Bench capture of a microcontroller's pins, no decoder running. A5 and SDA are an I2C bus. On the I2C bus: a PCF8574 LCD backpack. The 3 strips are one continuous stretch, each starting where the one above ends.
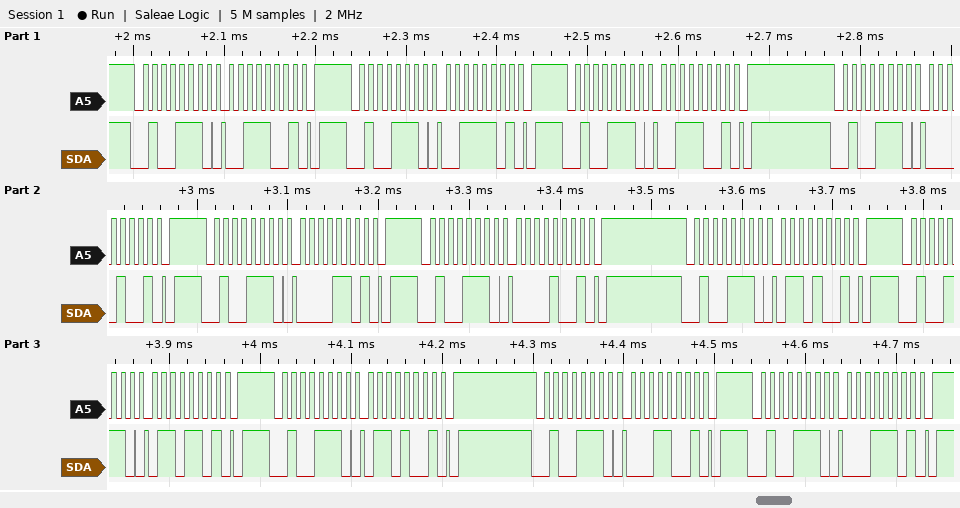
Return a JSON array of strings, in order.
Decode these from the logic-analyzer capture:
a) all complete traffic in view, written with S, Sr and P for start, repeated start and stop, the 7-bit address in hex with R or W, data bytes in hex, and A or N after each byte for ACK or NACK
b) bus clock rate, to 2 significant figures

["S 27W A 39 A P S 27W A 3D A P S 27W A 39 A P S 27W A 09 A P S 27W A 0D A P S 27W A 09 A P S 27W A 69 A P S 27W A 6D A P S 27W A 69 A P S 27W A 19 A P S 27W A 1D A P", "100 kHz"]
